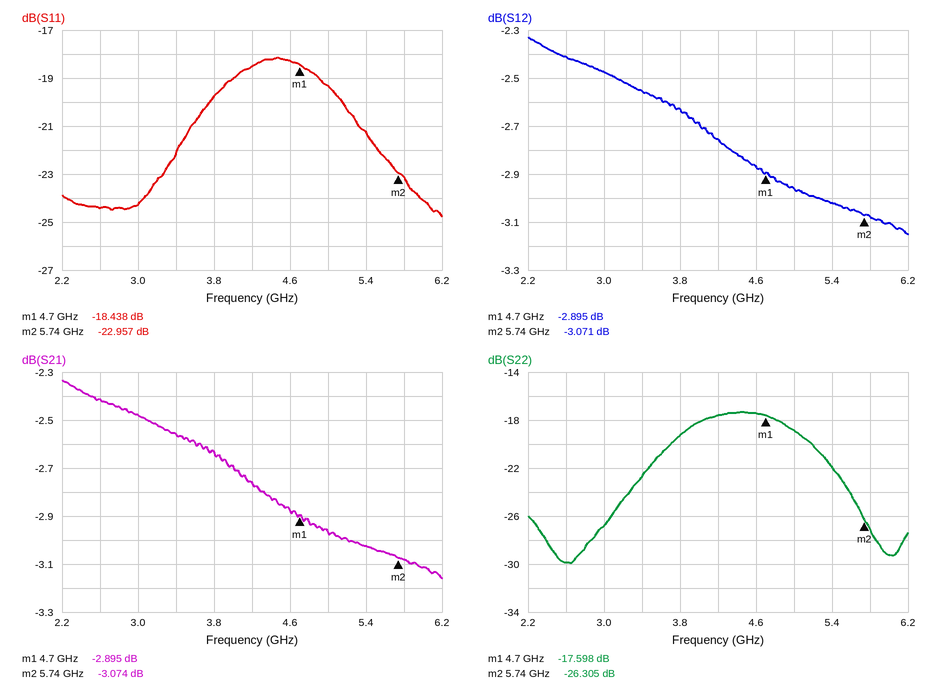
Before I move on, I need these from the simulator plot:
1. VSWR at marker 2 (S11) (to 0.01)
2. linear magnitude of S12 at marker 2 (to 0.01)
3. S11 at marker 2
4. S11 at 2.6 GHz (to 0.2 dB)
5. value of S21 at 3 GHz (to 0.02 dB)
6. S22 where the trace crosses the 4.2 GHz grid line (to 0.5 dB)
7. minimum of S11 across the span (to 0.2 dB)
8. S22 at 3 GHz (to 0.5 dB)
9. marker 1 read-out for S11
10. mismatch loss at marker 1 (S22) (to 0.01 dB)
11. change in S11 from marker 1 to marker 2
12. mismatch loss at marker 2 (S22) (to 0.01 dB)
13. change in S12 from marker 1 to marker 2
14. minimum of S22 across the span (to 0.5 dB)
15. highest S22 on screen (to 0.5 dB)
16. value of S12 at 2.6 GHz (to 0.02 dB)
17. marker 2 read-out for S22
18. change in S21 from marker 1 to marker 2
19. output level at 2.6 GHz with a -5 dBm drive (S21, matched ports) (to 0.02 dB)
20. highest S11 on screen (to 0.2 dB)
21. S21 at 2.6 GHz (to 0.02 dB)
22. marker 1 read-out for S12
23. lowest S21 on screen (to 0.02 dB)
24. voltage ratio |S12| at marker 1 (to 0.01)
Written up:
1.15
0.70
-22.957 dB
-24.4 dB
-2.48 dB
-17.5 dB
-24.8 dB
-27.0 dB
-18.438 dB
0.08 dB
-4.519 dB
0.01 dB
-0.176 dB
-30.0 dB
-17.5 dB
-2.42 dB
-26.305 dB
-0.179 dB
-7.42 dBm
-18.2 dB
-2.42 dB
-2.895 dB
-3.16 dB
0.72
